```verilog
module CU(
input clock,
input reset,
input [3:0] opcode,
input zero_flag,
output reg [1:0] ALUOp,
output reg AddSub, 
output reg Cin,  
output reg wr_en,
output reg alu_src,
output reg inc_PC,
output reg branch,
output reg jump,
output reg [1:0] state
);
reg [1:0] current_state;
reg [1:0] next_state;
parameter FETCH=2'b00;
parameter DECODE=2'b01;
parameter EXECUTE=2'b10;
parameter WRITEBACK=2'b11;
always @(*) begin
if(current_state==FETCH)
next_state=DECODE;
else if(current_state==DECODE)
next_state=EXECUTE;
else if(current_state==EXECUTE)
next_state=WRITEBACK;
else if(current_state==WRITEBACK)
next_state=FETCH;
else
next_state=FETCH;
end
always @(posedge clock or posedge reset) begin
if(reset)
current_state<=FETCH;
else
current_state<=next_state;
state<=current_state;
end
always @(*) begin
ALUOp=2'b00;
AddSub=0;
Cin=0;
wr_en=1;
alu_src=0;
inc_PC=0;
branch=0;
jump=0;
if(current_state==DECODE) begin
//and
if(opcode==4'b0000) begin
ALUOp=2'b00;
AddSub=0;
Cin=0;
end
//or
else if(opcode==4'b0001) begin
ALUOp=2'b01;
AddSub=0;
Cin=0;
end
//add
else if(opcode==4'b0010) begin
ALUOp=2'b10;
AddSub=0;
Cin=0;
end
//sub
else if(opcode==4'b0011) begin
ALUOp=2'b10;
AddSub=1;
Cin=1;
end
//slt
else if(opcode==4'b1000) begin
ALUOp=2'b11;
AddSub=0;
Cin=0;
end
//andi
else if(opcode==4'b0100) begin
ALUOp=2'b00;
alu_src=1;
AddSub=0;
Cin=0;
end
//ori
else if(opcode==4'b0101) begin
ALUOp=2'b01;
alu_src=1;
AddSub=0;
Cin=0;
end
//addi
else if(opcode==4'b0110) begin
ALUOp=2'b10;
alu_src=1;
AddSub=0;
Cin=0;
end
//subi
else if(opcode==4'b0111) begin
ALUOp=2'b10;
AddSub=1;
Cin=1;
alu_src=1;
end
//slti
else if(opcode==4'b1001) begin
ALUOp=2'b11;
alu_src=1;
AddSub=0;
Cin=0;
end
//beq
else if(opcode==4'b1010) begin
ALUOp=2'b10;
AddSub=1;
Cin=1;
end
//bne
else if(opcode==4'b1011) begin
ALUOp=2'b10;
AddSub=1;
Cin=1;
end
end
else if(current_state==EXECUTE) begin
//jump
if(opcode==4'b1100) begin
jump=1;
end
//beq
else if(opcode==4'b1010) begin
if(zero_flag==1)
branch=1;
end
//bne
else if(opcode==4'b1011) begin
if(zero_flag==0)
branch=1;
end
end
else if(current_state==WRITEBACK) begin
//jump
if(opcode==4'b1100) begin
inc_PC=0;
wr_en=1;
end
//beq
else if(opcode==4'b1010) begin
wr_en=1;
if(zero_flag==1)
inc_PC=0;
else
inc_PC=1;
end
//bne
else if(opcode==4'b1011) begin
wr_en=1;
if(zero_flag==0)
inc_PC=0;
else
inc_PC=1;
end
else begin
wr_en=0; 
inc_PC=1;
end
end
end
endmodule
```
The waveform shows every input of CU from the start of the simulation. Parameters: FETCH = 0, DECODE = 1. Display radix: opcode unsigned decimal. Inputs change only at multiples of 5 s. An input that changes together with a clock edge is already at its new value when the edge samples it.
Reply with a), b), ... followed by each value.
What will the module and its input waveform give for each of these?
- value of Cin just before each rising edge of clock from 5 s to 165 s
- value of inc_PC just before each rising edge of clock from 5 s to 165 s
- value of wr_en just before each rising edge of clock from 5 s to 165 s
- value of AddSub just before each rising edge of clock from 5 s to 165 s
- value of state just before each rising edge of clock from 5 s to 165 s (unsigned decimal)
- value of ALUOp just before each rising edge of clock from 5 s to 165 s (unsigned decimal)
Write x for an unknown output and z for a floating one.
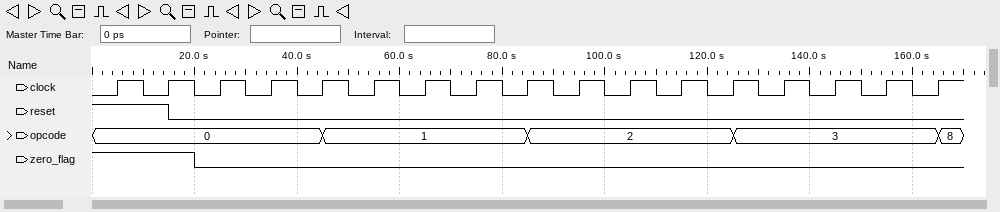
a) 0 0 0 0 0 0 0 0 0 0 0 0 0 0 1 0 0
b) 0 0 0 0 1 0 0 0 1 0 0 0 1 0 0 0 1
c) 1 1 1 1 0 1 1 1 0 1 1 1 0 1 1 1 0
d) 0 0 0 0 0 0 0 0 0 0 0 0 0 0 1 0 0
e) x, 0, 0, 1, 2, 3, 0, 1, 2, 3, 0, 1, 2, 3, 0, 1, 2
f) 0, 0, 0, 0, 0, 0, 1, 0, 0, 0, 2, 0, 0, 0, 2, 0, 0
